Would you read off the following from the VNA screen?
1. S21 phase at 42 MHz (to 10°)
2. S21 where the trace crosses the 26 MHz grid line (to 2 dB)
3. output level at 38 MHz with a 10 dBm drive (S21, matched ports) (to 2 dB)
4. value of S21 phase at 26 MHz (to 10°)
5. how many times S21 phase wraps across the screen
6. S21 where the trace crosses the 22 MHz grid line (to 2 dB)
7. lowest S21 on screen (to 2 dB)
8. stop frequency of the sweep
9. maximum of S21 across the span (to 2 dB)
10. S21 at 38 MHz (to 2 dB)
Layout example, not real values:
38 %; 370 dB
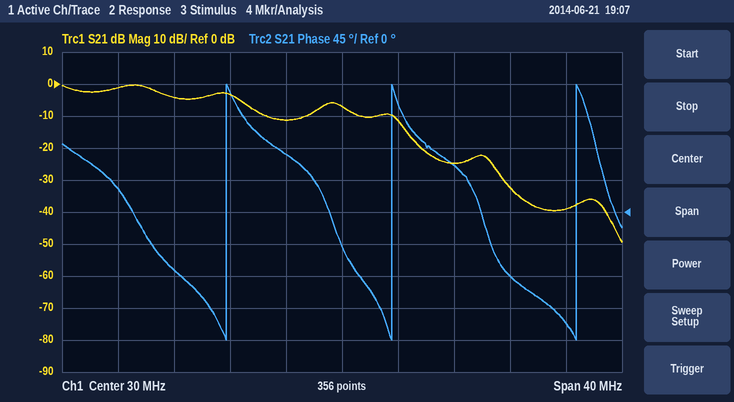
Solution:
-90°; -12 dB; -14 dBm; 80°; 3; -4 dB; -50 dB; 50 MHz; 0 dB; -24 dB
